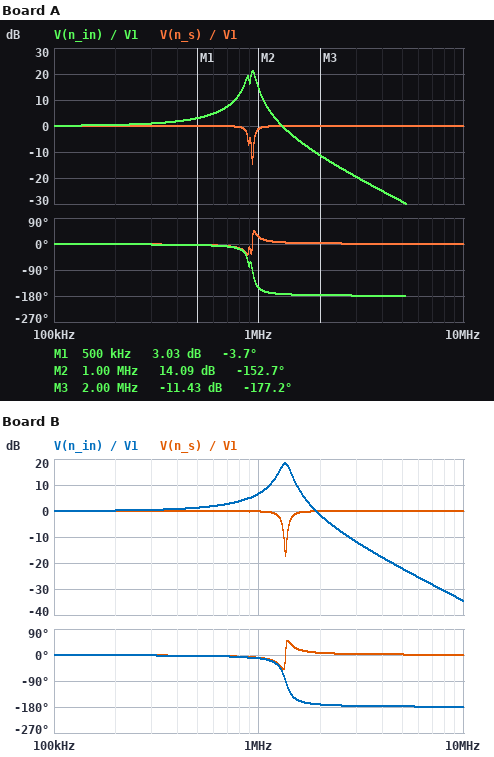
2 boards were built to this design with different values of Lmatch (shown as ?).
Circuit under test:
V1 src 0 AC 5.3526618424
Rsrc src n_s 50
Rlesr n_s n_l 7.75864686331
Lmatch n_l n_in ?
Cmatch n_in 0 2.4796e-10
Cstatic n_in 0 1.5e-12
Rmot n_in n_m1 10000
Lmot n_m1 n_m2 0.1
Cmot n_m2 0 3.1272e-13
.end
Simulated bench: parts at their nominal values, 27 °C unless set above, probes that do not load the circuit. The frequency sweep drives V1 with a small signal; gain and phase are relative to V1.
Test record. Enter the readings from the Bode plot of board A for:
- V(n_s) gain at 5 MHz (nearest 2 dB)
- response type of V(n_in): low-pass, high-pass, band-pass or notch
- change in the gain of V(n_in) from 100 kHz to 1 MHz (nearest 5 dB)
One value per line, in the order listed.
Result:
0 dB
low-pass
15 dB
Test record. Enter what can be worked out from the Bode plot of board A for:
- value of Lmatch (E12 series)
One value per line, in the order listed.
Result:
120 µH
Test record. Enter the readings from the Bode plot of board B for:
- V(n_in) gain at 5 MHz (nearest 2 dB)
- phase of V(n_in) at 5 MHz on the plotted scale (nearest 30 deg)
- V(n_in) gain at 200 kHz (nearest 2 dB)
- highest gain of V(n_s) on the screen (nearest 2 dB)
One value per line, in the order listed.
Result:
-22 dB
-180 deg
0 dB
0 dB
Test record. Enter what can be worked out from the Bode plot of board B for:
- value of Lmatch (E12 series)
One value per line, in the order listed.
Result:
56 µH
